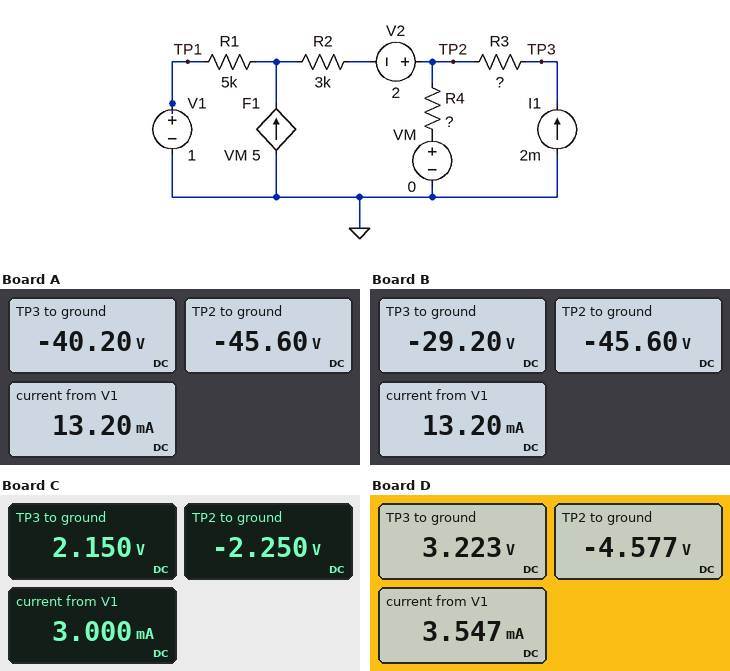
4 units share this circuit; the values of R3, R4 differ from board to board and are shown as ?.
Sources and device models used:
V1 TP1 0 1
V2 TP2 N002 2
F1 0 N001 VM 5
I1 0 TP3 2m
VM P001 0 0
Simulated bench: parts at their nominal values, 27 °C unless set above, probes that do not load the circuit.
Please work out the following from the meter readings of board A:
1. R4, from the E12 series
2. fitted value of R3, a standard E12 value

12 kΩ
2.7 kΩ
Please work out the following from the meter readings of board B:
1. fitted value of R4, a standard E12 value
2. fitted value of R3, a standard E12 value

12 kΩ
8.2 kΩ
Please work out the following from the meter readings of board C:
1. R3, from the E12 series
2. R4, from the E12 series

2.2 kΩ
1.8 kΩ
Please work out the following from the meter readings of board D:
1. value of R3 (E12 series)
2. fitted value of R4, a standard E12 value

3.9 kΩ
3.3 kΩ
